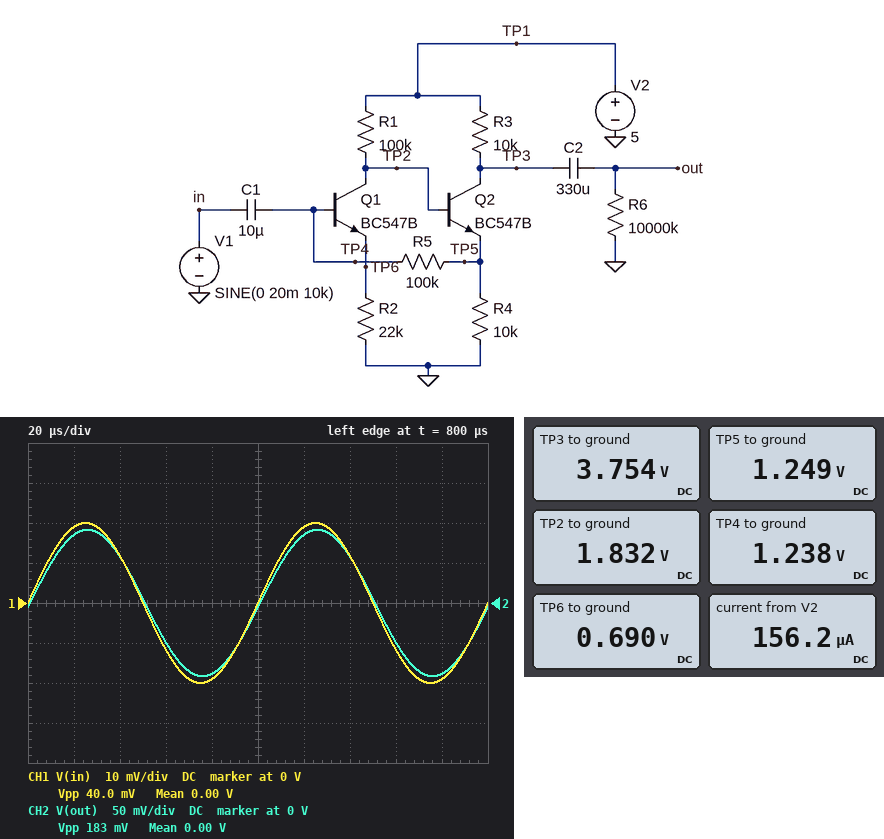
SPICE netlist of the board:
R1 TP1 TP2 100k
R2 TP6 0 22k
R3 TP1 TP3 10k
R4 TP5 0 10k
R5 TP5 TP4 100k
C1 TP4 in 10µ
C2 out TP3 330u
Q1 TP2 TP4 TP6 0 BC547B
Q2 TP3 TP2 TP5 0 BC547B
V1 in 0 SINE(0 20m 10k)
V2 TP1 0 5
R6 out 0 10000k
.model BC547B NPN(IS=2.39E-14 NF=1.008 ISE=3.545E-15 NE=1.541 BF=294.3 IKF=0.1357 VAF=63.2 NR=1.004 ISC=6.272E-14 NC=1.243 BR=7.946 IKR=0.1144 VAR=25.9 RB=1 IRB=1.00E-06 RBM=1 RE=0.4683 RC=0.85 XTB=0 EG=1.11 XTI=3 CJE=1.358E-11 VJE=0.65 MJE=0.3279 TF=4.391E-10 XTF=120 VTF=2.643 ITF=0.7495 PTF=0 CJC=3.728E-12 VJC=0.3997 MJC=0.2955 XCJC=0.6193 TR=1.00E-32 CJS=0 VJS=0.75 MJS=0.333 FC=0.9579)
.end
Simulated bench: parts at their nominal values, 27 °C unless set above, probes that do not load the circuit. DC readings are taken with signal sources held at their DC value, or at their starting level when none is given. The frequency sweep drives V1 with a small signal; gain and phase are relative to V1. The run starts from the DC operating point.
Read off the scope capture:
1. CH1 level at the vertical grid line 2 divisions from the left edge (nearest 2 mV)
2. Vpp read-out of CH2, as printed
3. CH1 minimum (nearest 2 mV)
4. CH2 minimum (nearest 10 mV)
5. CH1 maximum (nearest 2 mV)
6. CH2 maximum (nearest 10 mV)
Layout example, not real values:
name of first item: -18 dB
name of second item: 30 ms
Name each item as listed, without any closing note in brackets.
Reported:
CH1 level at the vertical grid line 2 divisions from the left edge: 12 mV
Vpp read-out of CH2, as printed: 183 mV
CH1 minimum: -20 mV
CH2 minimum: -90 mV
CH1 maximum: 20 mV
CH2 maximum: 90 mV
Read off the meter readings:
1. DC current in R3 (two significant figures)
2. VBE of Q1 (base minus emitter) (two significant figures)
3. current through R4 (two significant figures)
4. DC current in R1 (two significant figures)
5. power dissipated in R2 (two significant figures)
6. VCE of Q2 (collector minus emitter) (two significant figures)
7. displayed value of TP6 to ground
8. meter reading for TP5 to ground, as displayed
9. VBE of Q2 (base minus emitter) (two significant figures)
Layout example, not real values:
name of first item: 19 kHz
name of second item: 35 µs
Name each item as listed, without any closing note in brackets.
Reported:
DC current in R3: 120 µA
VBE of Q1 (base minus emitter): 550 mV
current through R4: 120 µA
DC current in R1: 32 µA
power dissipated in R2: 22 µW
VCE of Q2 (collector minus emitter): 2.5 V
displayed value of TP6 to ground: 0.690 V
meter reading for TP5 to ground, as displayed: 1.249 V
VBE of Q2 (base minus emitter): 580 mV
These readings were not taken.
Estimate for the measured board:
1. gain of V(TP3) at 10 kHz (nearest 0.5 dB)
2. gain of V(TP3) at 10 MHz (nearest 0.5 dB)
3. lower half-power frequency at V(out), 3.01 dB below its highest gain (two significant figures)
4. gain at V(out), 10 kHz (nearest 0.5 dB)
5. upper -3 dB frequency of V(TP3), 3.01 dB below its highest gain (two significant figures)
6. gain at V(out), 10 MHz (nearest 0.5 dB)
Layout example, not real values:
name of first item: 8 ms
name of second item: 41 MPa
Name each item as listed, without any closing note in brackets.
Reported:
gain of V(TP3) at 10 kHz: 13.0 dB
gain of V(TP3) at 10 MHz: -3.5 dB
lower half-power frequency at V(out), 3.01 dB below its highest gain: 810 mHz
gain at V(out), 10 kHz: 13.0 dB
upper -3 dB frequency of V(TP3), 3.01 dB below its highest gain: 200 kHz
gain at V(out), 10 MHz: -3.5 dB
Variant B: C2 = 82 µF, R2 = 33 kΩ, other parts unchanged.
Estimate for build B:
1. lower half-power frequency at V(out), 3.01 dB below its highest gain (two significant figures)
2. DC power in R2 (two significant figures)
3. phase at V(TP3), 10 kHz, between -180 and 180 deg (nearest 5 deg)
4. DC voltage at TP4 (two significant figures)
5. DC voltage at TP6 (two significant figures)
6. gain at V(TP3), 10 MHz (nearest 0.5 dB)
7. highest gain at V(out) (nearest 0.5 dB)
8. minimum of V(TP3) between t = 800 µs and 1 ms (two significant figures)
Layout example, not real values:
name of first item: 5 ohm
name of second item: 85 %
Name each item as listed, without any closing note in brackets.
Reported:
lower half-power frequency at V(out), 3.01 dB below its highest gain: 600 mHz
DC power in R2: 27 µW
phase at V(TP3), 10 kHz, between -180 and 180 deg: -5 deg
DC voltage at TP4: 1.5 V
DC voltage at TP6: 950 mV
gain at V(TP3), 10 MHz: -4.0 dB
highest gain at V(out): 10.0 dB
minimum of V(TP3) between t = 800 µs and 1 ms: 3.4 V
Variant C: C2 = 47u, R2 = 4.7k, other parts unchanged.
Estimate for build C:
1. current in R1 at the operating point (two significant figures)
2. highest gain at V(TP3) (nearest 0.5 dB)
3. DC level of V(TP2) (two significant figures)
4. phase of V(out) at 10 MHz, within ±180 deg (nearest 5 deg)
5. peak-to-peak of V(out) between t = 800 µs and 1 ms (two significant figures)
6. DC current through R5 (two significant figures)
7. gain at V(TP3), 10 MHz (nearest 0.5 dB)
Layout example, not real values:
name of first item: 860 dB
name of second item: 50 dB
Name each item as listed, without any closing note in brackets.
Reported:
current in R1 at the operating point: 37 µA
highest gain at V(TP3): 25.5 dB
DC level of V(TP2): 1.3 V
phase of V(out) at 10 MHz, within ±180 deg: 110 deg
peak-to-peak of V(out) between t = 800 µs and 1 ms: 740 mV
DC current through R5: 130 nA
gain at V(TP3), 10 MHz: -0.5 dB
